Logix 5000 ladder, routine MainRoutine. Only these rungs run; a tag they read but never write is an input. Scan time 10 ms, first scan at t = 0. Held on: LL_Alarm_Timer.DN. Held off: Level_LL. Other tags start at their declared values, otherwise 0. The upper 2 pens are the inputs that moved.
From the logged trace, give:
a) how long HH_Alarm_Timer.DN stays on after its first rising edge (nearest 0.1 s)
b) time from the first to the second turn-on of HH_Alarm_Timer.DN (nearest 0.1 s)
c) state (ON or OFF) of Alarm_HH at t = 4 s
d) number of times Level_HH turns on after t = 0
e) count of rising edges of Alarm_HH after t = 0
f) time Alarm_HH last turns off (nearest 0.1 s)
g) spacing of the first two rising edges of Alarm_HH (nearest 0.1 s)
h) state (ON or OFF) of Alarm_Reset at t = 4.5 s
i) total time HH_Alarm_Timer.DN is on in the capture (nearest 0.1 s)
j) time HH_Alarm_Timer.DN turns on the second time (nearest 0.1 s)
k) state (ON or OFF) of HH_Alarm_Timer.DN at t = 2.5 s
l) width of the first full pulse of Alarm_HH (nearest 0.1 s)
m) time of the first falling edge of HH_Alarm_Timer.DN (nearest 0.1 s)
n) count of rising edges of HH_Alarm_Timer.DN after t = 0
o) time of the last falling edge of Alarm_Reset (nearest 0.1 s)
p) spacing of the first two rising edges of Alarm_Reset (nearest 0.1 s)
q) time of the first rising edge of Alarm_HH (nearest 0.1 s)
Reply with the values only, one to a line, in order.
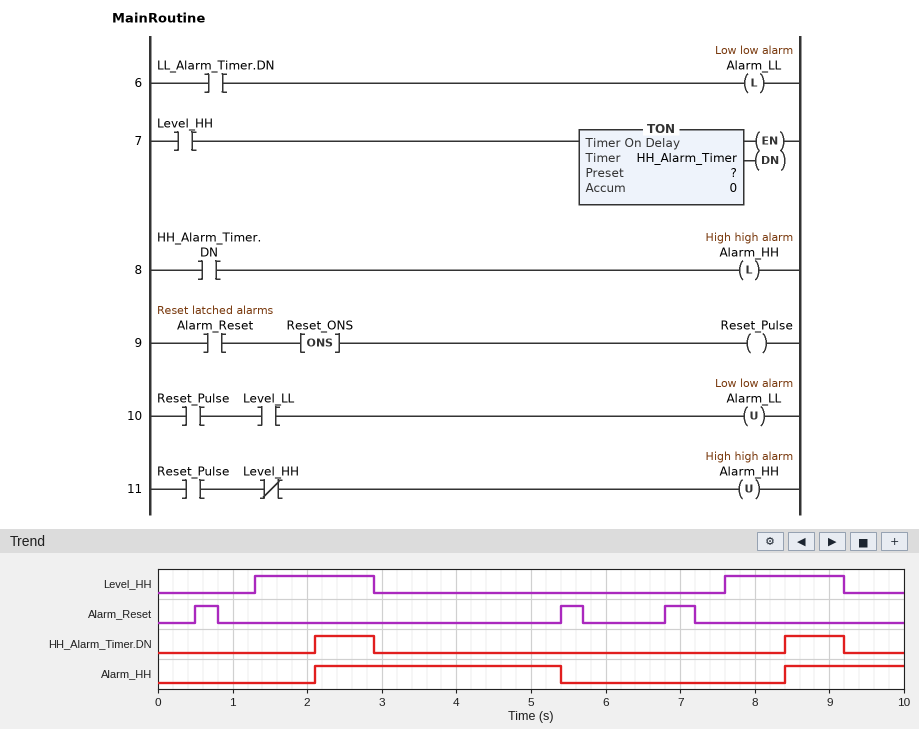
0.8 s
6.3 s
ON
2
2
5.4 s
6.3 s
OFF
1.6 s
8.4 s
ON
3.3 s
2.9 s
2
7.2 s
4.9 s
2.1 s
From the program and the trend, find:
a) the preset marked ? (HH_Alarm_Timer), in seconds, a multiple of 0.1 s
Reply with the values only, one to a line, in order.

0.8 s
